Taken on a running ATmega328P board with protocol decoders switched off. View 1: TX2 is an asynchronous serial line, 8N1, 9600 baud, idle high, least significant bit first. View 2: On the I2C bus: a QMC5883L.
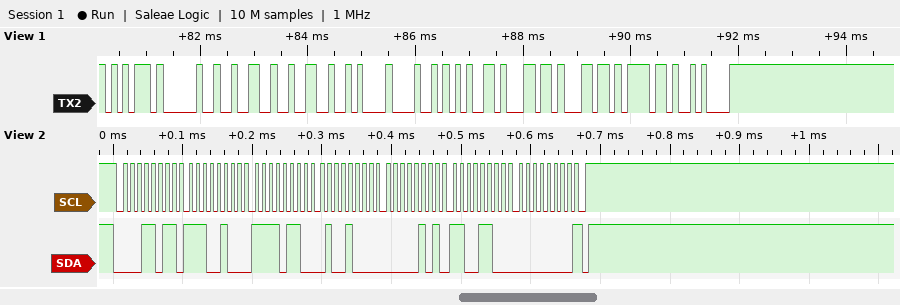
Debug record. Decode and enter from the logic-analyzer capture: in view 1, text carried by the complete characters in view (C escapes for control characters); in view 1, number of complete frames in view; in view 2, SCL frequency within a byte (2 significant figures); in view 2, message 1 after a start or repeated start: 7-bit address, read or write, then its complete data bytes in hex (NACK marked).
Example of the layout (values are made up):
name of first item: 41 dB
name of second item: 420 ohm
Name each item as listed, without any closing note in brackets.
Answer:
in view 1, text carried by the complete characters in view: "u 22\nHello\n"
in view 1, number of complete frames in view: 11
in view 2, SCL frequency within a byte: 100 kHz
in view 2, message 1 after a start or repeated start: 7-bit address, read or write, then its complete data bytes in hex: 0x0D read: E4 F6 48 05 CC 00 NACK
